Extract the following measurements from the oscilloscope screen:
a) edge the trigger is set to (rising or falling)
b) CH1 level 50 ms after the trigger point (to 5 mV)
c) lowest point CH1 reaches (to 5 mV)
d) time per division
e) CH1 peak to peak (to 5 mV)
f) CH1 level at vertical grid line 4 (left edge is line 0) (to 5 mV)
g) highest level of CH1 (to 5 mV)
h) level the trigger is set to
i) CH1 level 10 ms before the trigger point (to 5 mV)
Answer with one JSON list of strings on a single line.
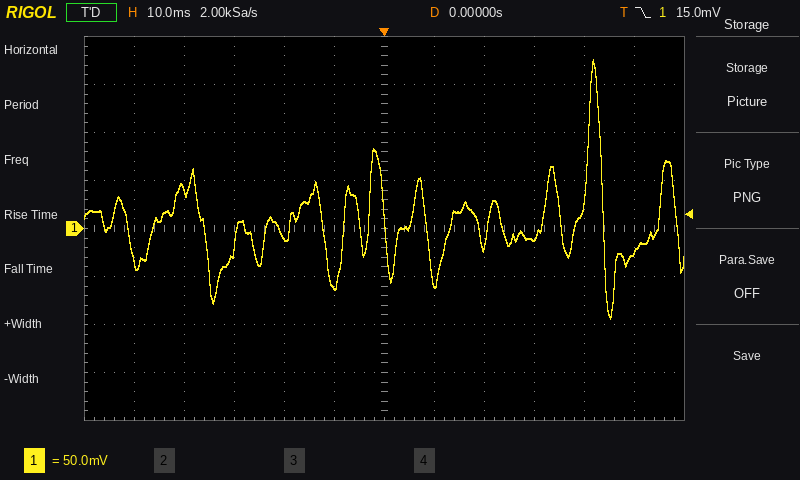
["falling", "-25 mV", "-95 mV", "10 ms", "270 mV", "-10 mV", "175 mV", "15.0 mV", "-60 mV"]
